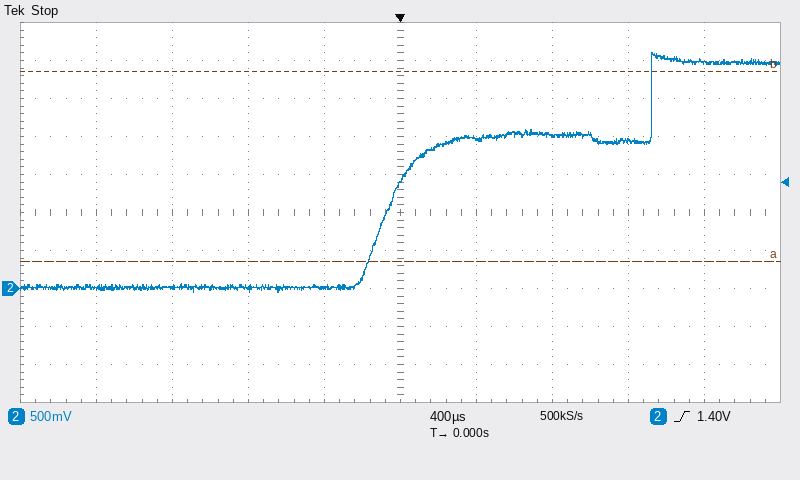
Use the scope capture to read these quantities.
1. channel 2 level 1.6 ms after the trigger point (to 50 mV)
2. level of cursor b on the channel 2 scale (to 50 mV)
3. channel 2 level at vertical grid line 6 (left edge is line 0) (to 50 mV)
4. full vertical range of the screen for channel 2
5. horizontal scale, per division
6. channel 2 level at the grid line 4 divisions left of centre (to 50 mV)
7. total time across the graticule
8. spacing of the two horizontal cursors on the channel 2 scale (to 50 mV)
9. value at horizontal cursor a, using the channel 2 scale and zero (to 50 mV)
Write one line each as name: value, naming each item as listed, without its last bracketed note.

channel 2 level 1.6 ms after the trigger point: 3.00 V
level of cursor b on the channel 2 scale: 2.85 V
channel 2 level at vertical grid line 6 (left edge is line 0): 1.95 V
full vertical range of the screen for channel 2: 5 V
horizontal scale, per division: 400 µs
channel 2 level at the grid line 4 divisions left of centre: 0 mV
total time across the graticule: 4 ms
spacing of the two horizontal cursors on the channel 2 scale: 2.50 V
value at horizontal cursor a, using the channel 2 scale and zero: 350 mV
